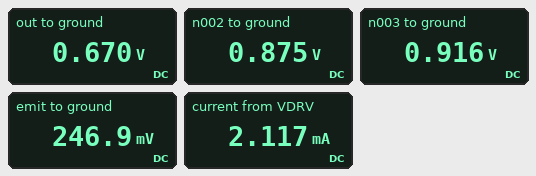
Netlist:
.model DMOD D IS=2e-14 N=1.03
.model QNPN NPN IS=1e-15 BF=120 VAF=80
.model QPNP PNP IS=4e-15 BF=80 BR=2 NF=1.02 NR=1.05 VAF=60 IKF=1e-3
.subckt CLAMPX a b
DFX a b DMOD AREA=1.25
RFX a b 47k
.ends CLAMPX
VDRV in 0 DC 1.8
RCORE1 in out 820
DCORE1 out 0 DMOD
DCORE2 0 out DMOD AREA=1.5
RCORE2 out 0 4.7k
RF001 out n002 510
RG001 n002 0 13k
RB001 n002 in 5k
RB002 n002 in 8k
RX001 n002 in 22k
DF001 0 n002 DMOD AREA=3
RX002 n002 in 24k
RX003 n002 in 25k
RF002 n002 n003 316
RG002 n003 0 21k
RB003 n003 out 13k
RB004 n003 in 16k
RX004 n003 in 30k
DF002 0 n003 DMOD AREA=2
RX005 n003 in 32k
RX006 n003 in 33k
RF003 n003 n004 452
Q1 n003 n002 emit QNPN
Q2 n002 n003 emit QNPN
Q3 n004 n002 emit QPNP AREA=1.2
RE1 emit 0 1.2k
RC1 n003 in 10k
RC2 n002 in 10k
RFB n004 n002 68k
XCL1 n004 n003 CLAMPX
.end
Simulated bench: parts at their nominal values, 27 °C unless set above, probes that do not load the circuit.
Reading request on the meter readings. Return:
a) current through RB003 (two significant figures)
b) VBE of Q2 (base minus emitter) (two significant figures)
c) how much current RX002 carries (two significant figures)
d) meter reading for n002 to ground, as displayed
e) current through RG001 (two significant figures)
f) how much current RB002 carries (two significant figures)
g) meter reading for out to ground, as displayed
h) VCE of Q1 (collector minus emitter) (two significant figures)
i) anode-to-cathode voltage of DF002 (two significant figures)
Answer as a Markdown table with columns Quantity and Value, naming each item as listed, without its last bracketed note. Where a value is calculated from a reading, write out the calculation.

| Quantity | Value |
|---|---|
| current through RB003 | (916 mV - 670 mV) / 13 kΩ = 19 µA |
| VBE of Q2 (base minus emitter) | 916 mV - 246.9 mV = 670 mV |
| how much current RX002 carries | (1.8 V - 875 mV) / 24 kΩ = 39 µA |
| meter reading for n002 to ground, as displayed | 0.875 V |
| current through RG001 | (875 mV) / 13 kΩ = 67 µA |
| how much current RB002 carries | (1.8 V - 875 mV) / 8 kΩ = 120 µA |
| meter reading for out to ground, as displayed | 0.670 V |
| VCE of Q1 (collector minus emitter) | 916 mV - 246.9 mV = 670 mV |
| anode-to-cathode voltage of DF002 | 0 V - 916 mV = -920 mV |
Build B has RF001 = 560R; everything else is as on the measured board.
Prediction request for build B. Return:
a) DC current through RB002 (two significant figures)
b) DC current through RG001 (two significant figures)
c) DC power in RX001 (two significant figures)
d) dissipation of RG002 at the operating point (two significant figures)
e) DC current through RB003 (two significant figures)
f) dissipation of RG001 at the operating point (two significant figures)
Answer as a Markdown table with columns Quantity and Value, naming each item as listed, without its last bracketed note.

| Quantity | Value |
|---|---|
| DC current through RB002 | 110 µA |
| DC current through RG001 | 68 µA |
| DC power in RX001 | 38 µW |
| dissipation of RG002 at the operating point | 41 µW |
| DC current through RB003 | 20 µA |
| dissipation of RG001 at the operating point | 60 µW |
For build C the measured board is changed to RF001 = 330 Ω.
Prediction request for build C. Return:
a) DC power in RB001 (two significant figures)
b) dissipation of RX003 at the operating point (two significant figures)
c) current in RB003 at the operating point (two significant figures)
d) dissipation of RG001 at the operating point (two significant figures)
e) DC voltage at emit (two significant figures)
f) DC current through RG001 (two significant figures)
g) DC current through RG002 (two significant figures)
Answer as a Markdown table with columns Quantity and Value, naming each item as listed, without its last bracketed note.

| Quantity | Value |
|---|---|
| DC power in RB001 | 190 µW |
| dissipation of RX003 at the operating point | 38 µW |
| current in RB003 at the operating point | 16 µA |
| dissipation of RG001 at the operating point | 53 µW |
| DC voltage at emit | 210 mV |
| DC current through RG001 | 64 µA |
| DC current through RG002 | 42 µA |
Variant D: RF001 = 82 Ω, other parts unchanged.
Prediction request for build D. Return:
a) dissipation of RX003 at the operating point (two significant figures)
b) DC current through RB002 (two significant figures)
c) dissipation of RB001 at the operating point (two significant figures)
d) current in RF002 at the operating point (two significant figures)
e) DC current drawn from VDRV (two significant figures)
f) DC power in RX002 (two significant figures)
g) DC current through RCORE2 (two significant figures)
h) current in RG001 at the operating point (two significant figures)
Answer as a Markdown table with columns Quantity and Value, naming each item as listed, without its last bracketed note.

| Quantity | Value |
|---|---|
| dissipation of RX003 at the operating point | 46 µW |
| DC current through RB002 | 130 µA |
| dissipation of RB001 at the operating point | 230 µW |
| current in RF002 at the operating point | 200 µA |
| DC current drawn from VDRV | 2.2 mA |
| DC power in RX002 | 48 µW |
| DC current through RCORE2 | 140 µA |
| current in RG001 at the operating point | 56 µA |
